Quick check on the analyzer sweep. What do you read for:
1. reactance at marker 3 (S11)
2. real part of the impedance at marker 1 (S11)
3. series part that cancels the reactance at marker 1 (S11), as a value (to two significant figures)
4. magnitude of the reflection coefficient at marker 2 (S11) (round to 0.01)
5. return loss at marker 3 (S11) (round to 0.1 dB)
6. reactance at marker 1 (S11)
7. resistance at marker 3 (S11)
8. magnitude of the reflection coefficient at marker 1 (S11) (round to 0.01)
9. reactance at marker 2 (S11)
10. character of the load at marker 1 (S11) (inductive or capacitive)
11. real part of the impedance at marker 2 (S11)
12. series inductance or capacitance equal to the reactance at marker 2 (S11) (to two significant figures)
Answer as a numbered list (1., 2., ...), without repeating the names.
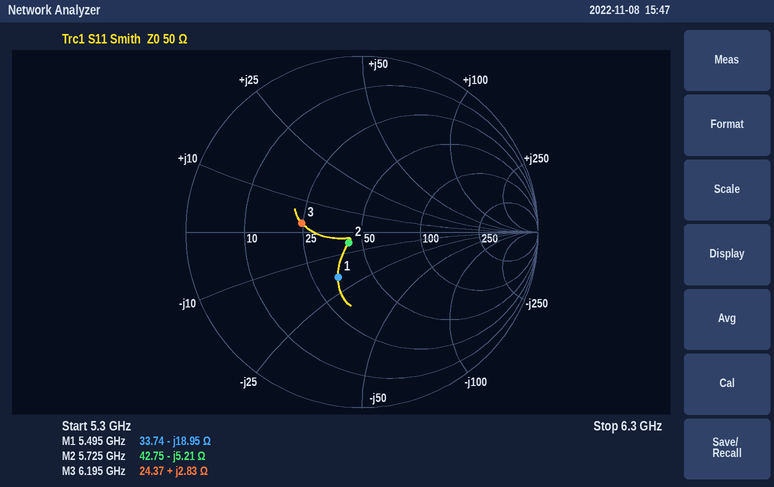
1. +2.83 Ω
2. 33.74 Ω
3. 550 pH
4. 0.10
5. 9.2 dB
6. -18.95 Ω
7. 24.37 Ω
8. 0.29
9. -5.21 Ω
10. capacitive
11. 42.75 Ω
12. 5.3 pF
